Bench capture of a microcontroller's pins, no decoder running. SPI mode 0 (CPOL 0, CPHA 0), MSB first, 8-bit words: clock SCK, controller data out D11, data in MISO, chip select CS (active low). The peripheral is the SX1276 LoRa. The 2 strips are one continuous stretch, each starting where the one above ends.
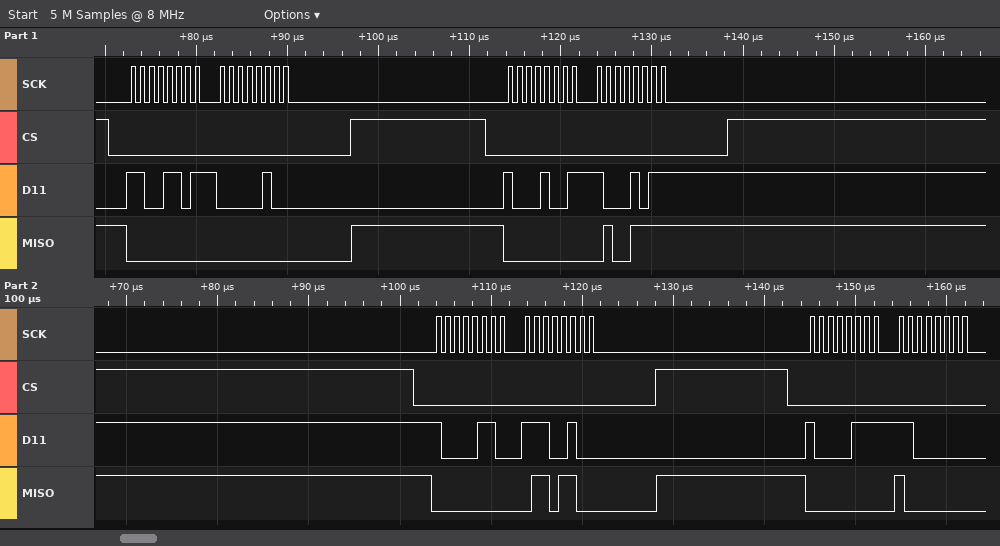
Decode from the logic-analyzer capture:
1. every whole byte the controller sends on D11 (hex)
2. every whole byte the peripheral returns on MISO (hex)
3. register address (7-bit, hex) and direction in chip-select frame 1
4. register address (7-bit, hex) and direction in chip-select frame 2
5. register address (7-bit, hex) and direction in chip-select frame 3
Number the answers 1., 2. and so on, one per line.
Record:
1. CD 04 89 8B 86 E4 87 C0
2. 00 00 00 4F 00 6C 00 80
3. 0x4D write
4. 0x09 write
5. 0x06 write
